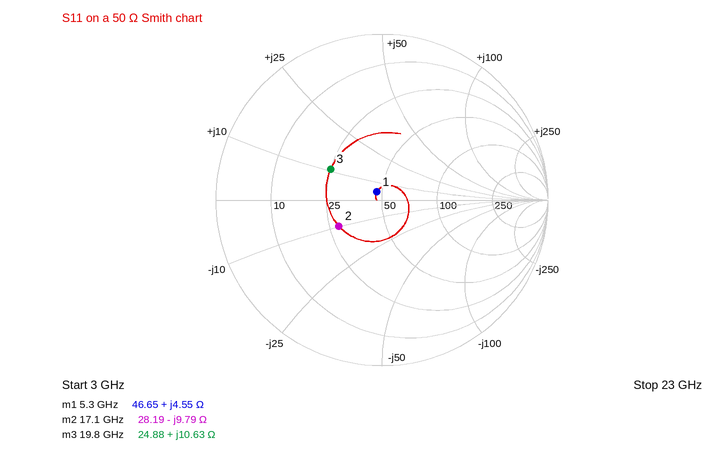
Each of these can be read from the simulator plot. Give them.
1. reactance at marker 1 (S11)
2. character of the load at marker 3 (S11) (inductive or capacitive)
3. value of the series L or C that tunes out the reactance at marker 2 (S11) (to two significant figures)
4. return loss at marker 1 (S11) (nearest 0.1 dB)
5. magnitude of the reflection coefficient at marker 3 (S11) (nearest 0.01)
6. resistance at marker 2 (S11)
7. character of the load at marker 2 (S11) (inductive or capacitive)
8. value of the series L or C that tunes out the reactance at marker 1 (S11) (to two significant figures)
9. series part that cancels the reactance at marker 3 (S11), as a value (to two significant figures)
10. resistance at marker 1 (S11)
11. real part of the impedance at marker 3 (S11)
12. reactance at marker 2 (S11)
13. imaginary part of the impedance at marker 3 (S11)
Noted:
+4.55 Ω
inductive
91 pH
24.7 dB
0.36
28.19 Ω
capacitive
6.6 pF
760 fF
46.65 Ω
24.88 Ω
-9.79 Ω
+10.63 Ω
